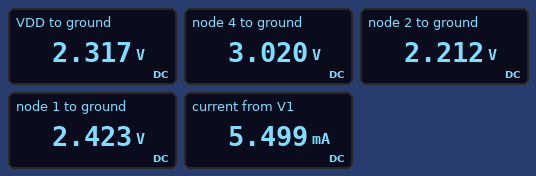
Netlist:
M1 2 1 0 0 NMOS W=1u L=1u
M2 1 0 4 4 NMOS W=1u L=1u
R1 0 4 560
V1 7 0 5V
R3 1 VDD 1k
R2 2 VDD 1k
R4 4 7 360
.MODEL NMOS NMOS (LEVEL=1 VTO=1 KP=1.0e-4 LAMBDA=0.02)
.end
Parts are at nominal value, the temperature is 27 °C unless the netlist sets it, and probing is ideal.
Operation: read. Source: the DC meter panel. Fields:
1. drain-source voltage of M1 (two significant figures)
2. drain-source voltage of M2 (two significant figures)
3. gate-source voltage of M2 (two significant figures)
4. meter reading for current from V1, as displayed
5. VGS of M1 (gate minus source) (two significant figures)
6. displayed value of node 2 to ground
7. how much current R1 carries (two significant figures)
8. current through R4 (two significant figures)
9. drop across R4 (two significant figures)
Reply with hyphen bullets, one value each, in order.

- 2.2 V
- -600 mV
- -3.0 V
- 5.499 mA
- 2.4 V
- 2.212 V
- 5.4 mA
- 5.5 mA
- 2.0 V
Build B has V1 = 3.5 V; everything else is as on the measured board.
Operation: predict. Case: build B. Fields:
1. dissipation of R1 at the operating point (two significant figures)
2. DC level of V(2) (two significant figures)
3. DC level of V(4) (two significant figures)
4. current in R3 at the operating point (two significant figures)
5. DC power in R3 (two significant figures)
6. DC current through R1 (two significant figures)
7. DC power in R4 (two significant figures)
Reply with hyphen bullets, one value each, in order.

- 8.1 mW
- 1.5 V
- 2.1 V
- 17 µA
- 290 nW
- 3.8 mA
- 5.2 mW
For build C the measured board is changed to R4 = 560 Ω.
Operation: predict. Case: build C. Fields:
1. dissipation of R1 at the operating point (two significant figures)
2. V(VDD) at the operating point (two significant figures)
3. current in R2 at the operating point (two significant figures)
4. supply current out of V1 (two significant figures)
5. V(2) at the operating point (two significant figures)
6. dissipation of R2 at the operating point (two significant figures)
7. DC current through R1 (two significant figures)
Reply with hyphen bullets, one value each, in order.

- 11 mW
- 1.9 V
- 43 µA
- 4.5 mA
- 1.8 V
- 1.9 µW
- 4.4 mA
